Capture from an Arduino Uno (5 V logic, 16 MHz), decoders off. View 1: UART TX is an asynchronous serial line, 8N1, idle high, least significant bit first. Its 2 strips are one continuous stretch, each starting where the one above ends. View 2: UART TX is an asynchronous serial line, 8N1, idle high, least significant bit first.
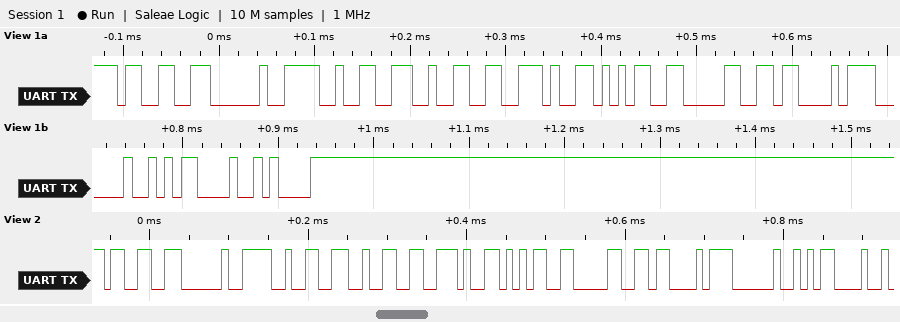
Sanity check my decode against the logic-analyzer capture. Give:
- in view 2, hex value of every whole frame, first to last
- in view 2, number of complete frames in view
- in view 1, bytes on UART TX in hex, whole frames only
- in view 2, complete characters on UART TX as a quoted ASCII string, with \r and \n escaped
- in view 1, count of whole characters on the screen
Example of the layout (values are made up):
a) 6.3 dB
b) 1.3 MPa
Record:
a) 0x33 0x20 0x32 0x32 0x2E 0x35 0x30 0x43 0x20 0x0D
b) 10
c) 0x33 0x20 0x32 0x32 0x2E 0x35 0x30 0x43 0x20 0x0D 0x0A
d) "3 22.50C \r"
e) 11
